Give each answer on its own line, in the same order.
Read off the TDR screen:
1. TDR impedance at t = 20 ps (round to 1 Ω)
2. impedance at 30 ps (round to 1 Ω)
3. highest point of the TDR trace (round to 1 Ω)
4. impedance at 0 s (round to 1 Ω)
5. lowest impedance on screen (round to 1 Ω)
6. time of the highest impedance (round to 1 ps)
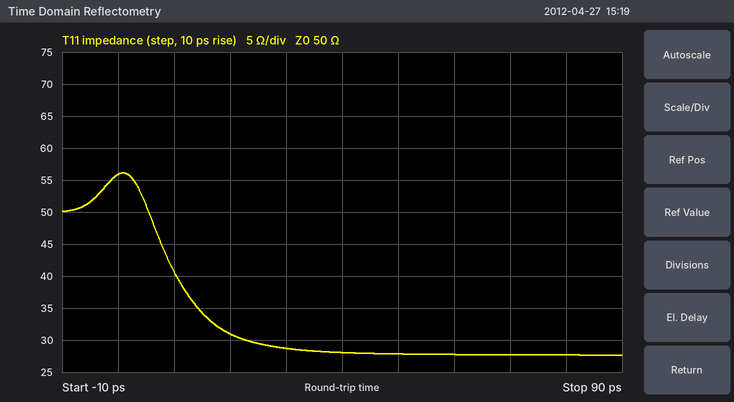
31 Ω
29 Ω
56 Ω
56 Ω
28 Ω
1 ps
